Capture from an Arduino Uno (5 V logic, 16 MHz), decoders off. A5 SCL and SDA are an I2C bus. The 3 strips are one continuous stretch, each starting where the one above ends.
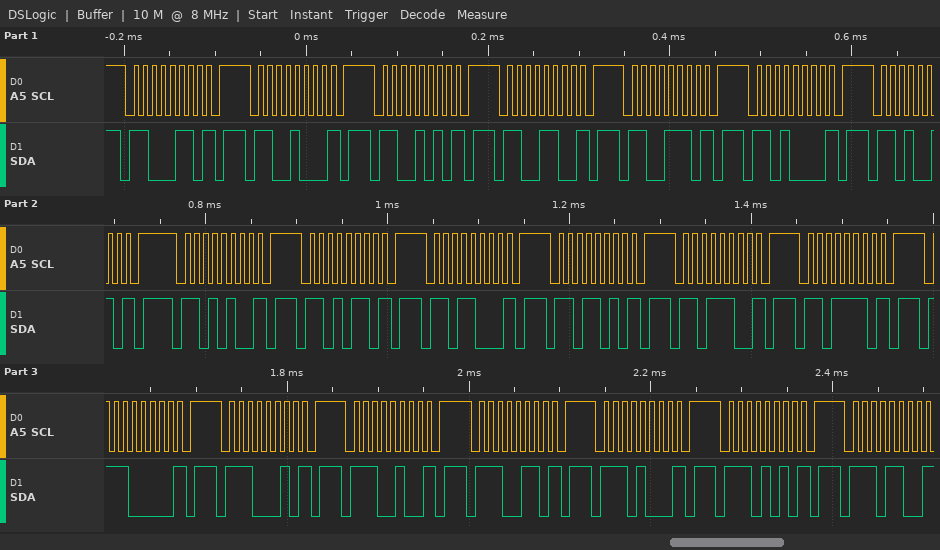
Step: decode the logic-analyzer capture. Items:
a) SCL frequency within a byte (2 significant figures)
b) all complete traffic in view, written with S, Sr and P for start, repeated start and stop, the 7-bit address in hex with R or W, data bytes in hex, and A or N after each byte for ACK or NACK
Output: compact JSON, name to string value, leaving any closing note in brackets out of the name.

{"SCL frequency within a byte": "100 kHz", "all complete traffic in view, written with S, Sr and P for start, repeated start and stop, the 7-bit address in hex with R or W, data bytes in hex, and A or N after each byte for ACK or NACK": "S 63W N P S 64W N P S 65W N P S 66W N P S 67W N P S 68W N P S 69W N P S 6AW N P S 6BW N P S 6CW N P S 6DW N P S 6EW N P S 6FW N P S 70W N P S 71W N P S 72W N P S 73W N P S 74W N P S 75W N P S 76W N"}
